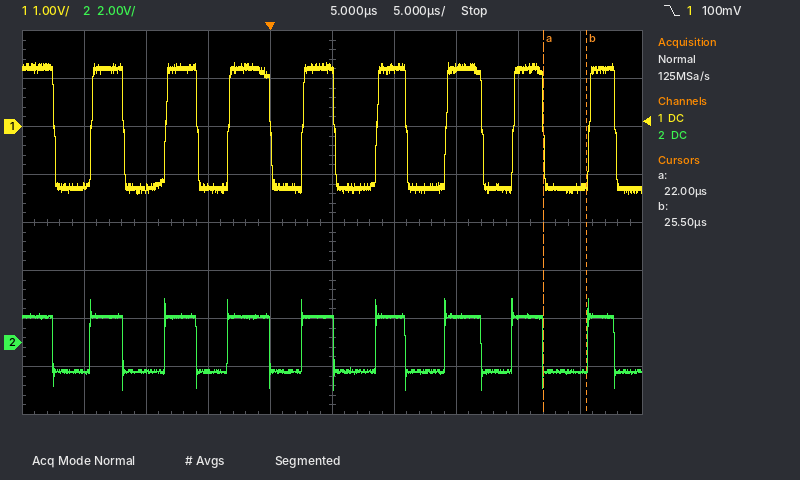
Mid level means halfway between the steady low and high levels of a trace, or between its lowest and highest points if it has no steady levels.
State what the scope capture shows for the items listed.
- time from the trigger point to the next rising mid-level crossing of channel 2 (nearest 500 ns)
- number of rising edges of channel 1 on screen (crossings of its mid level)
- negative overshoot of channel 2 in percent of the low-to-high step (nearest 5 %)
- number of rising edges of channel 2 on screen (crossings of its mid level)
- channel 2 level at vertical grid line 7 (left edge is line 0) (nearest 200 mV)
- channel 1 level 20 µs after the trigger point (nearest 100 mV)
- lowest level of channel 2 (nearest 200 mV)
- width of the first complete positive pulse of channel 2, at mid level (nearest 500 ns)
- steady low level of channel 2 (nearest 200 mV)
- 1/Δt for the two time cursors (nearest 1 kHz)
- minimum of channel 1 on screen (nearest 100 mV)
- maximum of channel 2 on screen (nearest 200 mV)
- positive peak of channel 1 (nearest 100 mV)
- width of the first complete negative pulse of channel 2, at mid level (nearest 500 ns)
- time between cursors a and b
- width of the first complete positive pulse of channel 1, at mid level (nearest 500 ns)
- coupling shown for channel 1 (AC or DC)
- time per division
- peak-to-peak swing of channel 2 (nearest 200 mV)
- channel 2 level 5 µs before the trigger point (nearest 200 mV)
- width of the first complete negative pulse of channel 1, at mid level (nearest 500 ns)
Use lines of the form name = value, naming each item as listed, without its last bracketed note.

time from the trigger point to the next rising mid-level crossing of channel 2 = 2.5 µs
number of rising edges of channel 1 on screen = 8
negative overshoot of channel 2 in percent of the low-to-high step = 35 %
number of rising edges of channel 2 on screen = 8
channel 2 level at vertical grid line 7 (left edge is line 0) = 1.0 V
channel 1 level 20 µs after the trigger point = 1.2 V
lowest level of channel 2 = -2.0 V
width of the first complete positive pulse of channel 2, at mid level = 2.5 µs
steady low level of channel 2 = -1.2 V
1/Δt for the two time cursors = 286 kHz
minimum of channel 1 on screen = -1.4 V
maximum of channel 2 on screen = 1.8 V
positive peak of channel 1 = 1.3 V
width of the first complete negative pulse of channel 2, at mid level = 3.0 µs
time between cursors a and b = 3.5 µs
width of the first complete positive pulse of channel 1, at mid level = 2.5 µs
coupling shown for channel 1 = DC
time per division = 5 µs
peak-to-peak swing of channel 2 = 3.8 V
channel 2 level 5 µs before the trigger point = -1.2 V
width of the first complete negative pulse of channel 1, at mid level = 3.0 µs
